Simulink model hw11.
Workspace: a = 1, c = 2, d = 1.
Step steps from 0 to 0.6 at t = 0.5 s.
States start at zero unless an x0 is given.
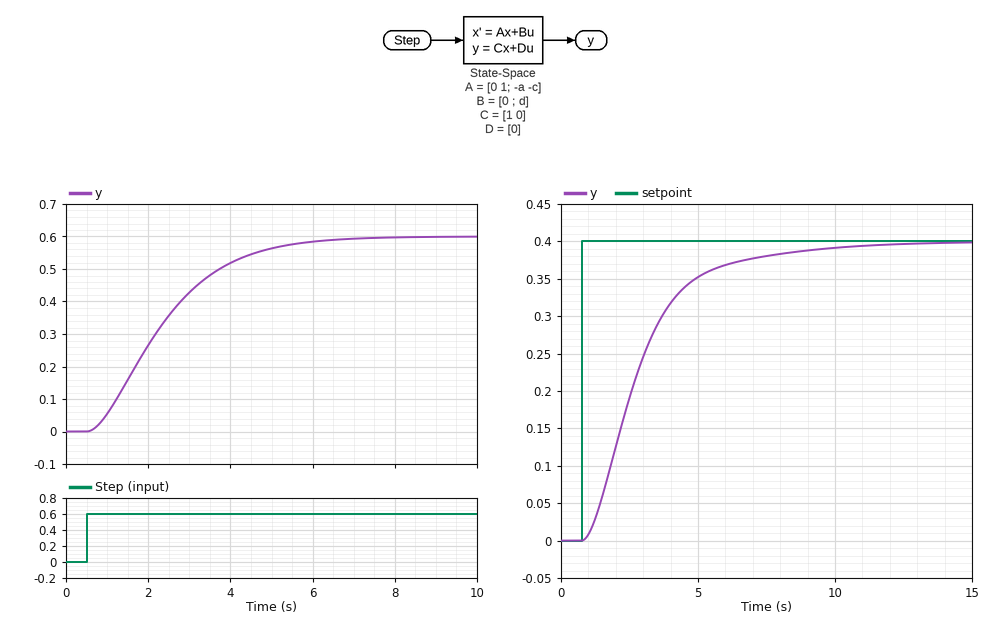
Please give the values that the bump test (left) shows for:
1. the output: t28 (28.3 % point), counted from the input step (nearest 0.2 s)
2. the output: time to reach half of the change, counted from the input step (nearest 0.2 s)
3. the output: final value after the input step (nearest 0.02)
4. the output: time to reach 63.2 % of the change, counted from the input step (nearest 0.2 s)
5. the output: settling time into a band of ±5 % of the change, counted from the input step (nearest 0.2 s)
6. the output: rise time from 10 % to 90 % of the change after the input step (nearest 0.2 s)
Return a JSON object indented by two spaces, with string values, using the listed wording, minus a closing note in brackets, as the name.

{
  "the output: t28 (28.3 % point), counted from the input step": "1.0 s",
  "the output: time to reach half of the change, counted from the input step": "1.6 s",
  "the output: final value after the input step": "0.60",
  "the output: time to reach 63.2 % of the change, counted from the input step": "2.2 s",
  "the output: settling time into a band of ±5 % of the change, counted from the input step": "4.8 s",
  "the output: rise time from 10 % to 90 % of the change after the input step": "3.4 s"
}
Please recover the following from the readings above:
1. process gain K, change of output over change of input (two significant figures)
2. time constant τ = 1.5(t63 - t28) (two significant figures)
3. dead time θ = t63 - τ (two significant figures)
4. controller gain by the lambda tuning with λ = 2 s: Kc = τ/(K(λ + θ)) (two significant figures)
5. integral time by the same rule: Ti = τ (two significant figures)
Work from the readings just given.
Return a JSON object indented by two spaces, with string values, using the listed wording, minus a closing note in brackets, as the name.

{
  "process gain K, change of output over change of input": "1.0",
  "time constant τ = 1.5(t63 - t28)": "1.8 s",
  "dead time θ = t63 - τ": "0.40 s",
  "controller gain by the lambda tuning with λ = 2 s: Kc = τ/(K(λ + θ))": "0.75",
  "integral time by the same rule: Ti = τ": "1.8 s"
}
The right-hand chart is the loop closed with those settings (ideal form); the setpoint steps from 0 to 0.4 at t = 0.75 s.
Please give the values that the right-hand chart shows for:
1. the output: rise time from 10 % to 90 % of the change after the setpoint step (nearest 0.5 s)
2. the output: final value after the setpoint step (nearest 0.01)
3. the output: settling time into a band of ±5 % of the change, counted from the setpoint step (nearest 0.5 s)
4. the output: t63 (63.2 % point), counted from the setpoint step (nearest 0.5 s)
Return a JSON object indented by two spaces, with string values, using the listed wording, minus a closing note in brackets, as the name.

{
  "the output: rise time from 10 % to 90 % of the change after the setpoint step": "4.0 s",
  "the output: final value after the setpoint step": "0.40",
  "the output: settling time into a band of ±5 % of the change, counted from the setpoint step": "6.5 s",
  "the output: t63 (63.2 % point), counted from the setpoint step": "2.5 s"
}
